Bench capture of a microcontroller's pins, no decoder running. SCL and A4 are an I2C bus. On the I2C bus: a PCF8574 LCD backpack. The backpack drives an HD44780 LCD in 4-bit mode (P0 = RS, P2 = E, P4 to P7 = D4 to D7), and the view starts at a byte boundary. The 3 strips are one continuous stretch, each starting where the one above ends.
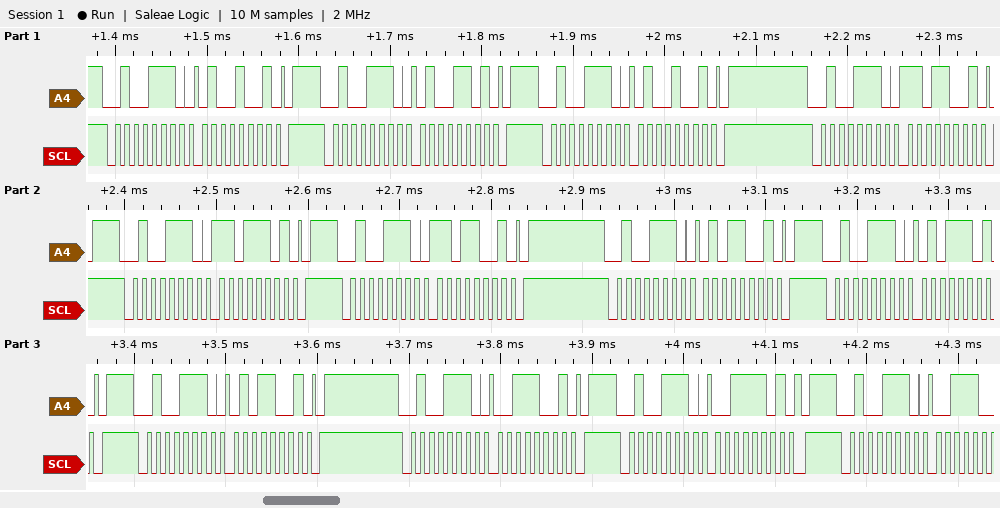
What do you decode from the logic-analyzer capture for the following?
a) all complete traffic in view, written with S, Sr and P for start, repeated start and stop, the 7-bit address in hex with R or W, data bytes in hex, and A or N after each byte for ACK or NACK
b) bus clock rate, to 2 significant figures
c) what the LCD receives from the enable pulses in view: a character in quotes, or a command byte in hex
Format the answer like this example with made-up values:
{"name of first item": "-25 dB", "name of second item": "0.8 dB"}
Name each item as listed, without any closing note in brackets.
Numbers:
{"all complete traffic in view, written with S, Sr and P for start, repeated start and stop, the 7-bit address in hex with R or W, data bytes in hex, and A or N after each byte for ACK or NACK": "S 27W A 49 A P S 27W A 4D A P S 27W A 49 A P S 27W A D9 A P S 27W A DD A P S 27W A D9 A P S 27W A 59 A P S 27W A 5D A P S 27W A 59 A P S 27W A 39 A P S 27W A 3D A P S 27W A", "bus clock rate, to 2 significant figures": "100 kHz", "what the LCD receives from the enable pulses in view: a character in quotes, or a command byte in hex": "'M'"}
